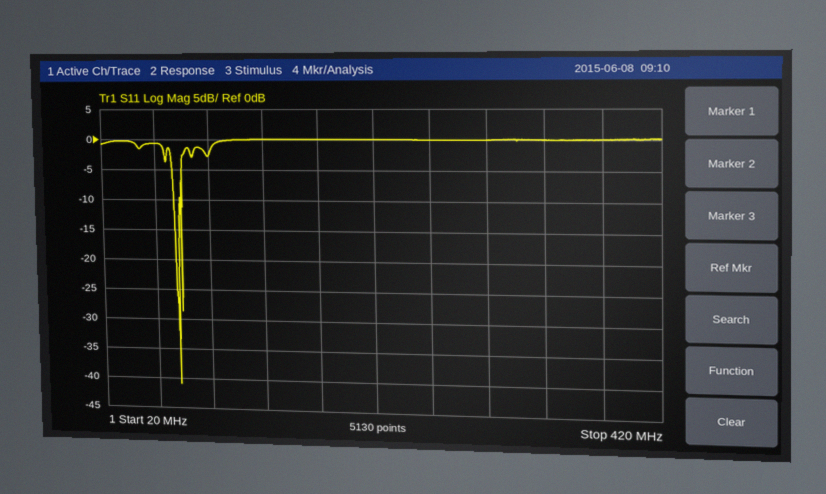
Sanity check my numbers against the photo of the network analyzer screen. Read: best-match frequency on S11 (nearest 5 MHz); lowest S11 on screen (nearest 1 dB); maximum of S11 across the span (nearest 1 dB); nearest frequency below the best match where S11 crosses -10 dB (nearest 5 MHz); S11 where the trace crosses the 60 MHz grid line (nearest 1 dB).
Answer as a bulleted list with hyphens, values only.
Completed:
- 75 MHz
- -41 dB
- 0 dB
- 75 MHz
- -1 dB
